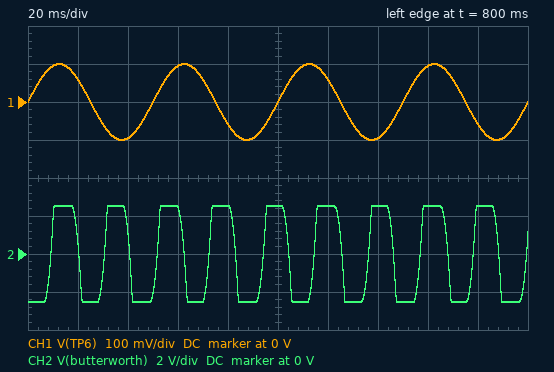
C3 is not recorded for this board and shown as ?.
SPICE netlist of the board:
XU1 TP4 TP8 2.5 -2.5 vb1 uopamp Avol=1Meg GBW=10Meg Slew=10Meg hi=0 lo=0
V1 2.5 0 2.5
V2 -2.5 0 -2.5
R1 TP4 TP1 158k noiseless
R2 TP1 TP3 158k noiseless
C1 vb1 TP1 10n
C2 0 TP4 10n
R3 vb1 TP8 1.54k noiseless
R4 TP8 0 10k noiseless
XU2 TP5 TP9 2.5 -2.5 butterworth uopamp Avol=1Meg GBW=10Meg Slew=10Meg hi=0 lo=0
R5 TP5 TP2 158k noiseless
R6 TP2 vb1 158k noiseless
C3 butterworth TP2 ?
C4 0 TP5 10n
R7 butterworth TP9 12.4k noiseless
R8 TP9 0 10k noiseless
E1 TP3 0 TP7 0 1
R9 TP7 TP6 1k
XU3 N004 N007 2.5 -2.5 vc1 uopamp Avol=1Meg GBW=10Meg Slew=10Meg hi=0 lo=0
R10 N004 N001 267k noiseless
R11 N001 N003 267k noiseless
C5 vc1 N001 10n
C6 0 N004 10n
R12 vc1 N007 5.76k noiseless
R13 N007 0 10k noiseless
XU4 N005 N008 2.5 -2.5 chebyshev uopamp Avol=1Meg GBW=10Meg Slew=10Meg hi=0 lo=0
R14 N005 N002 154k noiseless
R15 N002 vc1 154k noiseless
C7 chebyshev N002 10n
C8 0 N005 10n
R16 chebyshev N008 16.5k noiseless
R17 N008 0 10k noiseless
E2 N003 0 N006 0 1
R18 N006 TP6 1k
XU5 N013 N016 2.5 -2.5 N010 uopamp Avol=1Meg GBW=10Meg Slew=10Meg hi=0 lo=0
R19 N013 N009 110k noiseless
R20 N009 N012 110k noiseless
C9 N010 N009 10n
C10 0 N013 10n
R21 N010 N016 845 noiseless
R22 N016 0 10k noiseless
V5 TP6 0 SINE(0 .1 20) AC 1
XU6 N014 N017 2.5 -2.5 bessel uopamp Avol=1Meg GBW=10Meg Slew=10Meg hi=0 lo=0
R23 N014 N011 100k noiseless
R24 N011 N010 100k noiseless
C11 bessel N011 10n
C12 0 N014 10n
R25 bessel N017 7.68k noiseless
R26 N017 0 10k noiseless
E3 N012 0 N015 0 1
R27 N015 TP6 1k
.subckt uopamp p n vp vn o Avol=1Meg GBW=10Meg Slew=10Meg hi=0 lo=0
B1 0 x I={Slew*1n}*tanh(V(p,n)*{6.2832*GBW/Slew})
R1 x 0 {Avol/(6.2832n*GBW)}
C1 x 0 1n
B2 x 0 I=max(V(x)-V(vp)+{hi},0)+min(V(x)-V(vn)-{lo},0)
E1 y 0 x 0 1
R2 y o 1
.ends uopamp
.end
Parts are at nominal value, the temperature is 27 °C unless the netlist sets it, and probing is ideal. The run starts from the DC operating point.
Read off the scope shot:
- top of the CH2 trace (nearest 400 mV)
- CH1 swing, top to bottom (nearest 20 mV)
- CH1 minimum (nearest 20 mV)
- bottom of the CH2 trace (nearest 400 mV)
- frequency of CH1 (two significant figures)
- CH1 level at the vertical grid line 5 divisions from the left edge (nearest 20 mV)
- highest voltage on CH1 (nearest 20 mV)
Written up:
2.4 V
200 mV
-100 mV
-2.4 V
20 Hz
0 V
100 mV
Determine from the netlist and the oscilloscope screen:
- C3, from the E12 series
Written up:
33 nF
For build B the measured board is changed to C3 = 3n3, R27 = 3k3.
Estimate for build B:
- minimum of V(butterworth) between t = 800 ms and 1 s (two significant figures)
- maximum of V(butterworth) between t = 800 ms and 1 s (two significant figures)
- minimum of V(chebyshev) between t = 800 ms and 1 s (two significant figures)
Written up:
-240 mV
240 mV
-430 mV
